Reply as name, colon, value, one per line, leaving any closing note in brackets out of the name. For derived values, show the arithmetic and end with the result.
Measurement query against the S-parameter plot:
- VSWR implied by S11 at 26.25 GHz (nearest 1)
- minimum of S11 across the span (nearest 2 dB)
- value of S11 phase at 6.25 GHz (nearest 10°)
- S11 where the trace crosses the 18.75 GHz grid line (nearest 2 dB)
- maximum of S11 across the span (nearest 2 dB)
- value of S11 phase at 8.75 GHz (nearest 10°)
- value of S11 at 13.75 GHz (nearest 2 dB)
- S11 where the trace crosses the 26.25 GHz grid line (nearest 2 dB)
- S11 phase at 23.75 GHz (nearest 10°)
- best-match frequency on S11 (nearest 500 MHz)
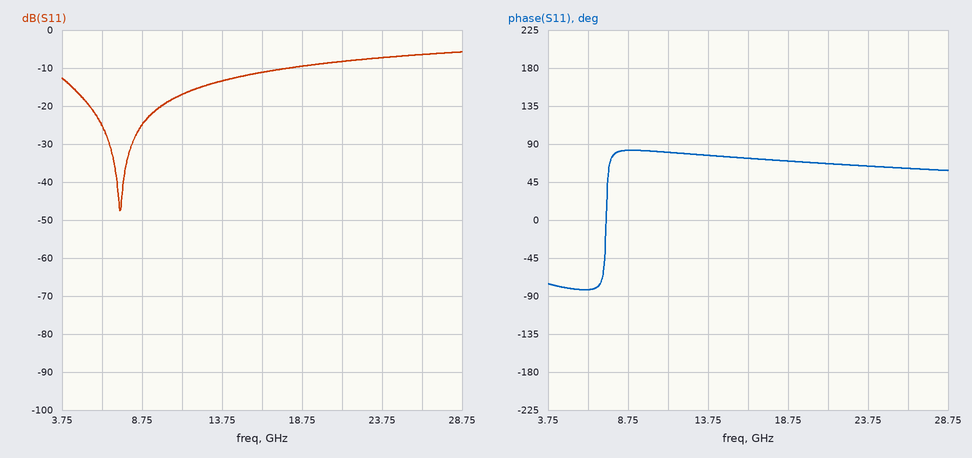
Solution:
VSWR implied by S11 at 26.25 GHz: |Γ| = 10^(-6/20) = 0.5012; VSWR = (1 + 0.5012)/(1 − 0.5012) ≈ 3
minimum of S11 across the span: -48 dB
value of S11 phase at 6.25 GHz: -80°
S11 where the trace crosses the 18.75 GHz grid line: -10 dB
maximum of S11 across the span: -6 dB
value of S11 phase at 8.75 GHz: 80°
value of S11 at 13.75 GHz: -14 dB
S11 where the trace crosses the 26.25 GHz grid line: -6 dB
S11 phase at 23.75 GHz: 60°
best-match frequency on S11: 7.5 GHz
